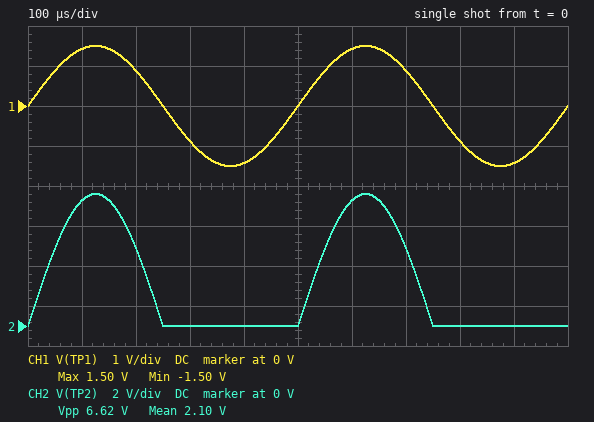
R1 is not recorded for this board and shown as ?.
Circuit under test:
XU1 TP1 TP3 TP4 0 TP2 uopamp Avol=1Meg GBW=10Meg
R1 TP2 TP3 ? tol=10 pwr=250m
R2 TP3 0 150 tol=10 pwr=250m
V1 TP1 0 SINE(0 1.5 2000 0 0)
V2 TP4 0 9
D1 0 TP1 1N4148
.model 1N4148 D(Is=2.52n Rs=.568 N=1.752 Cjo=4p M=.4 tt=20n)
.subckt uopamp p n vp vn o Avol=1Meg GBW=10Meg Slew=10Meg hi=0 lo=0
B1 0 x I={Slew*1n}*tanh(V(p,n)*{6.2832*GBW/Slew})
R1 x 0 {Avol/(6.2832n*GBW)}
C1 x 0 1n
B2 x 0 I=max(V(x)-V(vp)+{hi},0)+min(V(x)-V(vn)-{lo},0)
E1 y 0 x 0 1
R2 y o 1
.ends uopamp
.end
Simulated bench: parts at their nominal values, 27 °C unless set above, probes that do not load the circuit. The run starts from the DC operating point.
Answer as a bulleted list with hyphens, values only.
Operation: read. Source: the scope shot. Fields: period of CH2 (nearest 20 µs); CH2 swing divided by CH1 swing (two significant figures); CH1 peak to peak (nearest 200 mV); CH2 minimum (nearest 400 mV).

- 500 µs
- 2.2
- 3.0 V
- 0 V
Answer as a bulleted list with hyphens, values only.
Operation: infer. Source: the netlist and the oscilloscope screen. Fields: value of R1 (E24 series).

- 510 Ω
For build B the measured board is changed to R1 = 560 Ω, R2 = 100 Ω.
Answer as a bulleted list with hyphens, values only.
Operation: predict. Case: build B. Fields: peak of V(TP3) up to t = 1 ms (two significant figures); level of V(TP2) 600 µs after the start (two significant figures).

- 1.4 V
- 9.0 V
